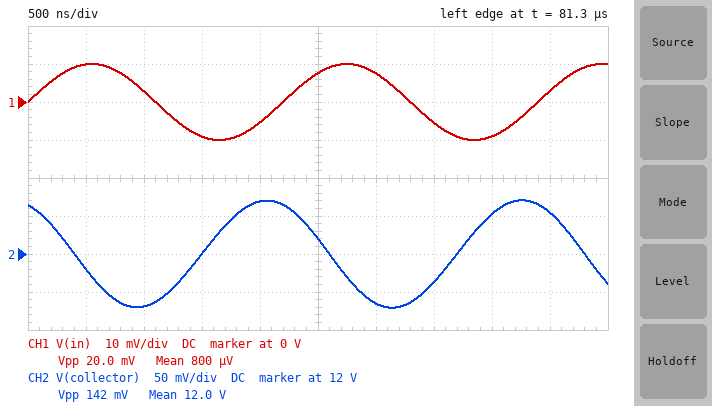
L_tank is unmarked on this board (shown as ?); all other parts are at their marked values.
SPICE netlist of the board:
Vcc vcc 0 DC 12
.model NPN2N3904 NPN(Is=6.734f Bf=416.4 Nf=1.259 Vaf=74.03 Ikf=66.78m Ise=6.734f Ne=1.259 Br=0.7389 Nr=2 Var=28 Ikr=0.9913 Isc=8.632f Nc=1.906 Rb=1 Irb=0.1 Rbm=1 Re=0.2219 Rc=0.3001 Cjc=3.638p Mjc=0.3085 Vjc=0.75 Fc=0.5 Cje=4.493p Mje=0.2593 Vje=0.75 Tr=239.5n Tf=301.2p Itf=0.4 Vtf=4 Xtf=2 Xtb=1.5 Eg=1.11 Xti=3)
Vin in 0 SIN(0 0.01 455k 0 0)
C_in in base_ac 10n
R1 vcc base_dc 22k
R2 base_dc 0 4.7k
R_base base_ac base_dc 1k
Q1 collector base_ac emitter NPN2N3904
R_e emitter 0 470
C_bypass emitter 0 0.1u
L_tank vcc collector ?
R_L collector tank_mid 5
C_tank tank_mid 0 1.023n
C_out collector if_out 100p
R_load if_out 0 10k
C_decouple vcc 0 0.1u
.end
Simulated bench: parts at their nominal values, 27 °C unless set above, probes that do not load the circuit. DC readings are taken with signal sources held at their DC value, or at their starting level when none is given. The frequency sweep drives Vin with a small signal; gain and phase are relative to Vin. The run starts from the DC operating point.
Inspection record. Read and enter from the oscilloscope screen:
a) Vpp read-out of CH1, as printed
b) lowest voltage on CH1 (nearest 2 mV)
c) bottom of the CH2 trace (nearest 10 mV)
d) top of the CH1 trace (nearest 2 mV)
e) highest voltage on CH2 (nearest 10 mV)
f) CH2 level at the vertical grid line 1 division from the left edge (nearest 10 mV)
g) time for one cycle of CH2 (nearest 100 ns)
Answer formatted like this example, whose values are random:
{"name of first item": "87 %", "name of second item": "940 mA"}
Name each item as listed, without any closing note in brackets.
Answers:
{"Vpp read-out of CH1, as printed": "20.0 mV", "lowest voltage on CH1": "-10 mV", "bottom of the CH2 trace": "11.93 V", "top of the CH1 trace": "10 mV", "highest voltage on CH2": "12.07 V", "CH2 level at the vertical grid line 1 division from the left edge": "11.98 V", "time for one cycle of CH2": "2.2 µs"}
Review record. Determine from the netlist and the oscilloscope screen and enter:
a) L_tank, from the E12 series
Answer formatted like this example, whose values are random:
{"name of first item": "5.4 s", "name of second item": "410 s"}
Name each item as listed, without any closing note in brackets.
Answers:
{"L_tank, from the E12 series": "180 µH"}
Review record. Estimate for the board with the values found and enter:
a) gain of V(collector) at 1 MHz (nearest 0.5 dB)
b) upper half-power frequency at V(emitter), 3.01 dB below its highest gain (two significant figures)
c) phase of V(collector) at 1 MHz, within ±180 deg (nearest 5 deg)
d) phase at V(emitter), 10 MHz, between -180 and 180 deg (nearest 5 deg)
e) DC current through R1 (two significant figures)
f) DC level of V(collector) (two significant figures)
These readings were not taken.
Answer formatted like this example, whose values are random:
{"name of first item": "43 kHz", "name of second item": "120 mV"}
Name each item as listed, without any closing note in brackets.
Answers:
{"gain of V(collector) at 1 MHz": "2.5 dB", "upper half-power frequency at V(emitter), 3.01 dB below its highest gain": "140 kHz", "phase of V(collector) at 1 MHz, within ±180 deg": "100 deg", "phase at V(emitter), 10 MHz, between -180 and 180 deg": "-85 deg", "DC current through R1": "490 µA", "DC level of V(collector)": "12 V"}
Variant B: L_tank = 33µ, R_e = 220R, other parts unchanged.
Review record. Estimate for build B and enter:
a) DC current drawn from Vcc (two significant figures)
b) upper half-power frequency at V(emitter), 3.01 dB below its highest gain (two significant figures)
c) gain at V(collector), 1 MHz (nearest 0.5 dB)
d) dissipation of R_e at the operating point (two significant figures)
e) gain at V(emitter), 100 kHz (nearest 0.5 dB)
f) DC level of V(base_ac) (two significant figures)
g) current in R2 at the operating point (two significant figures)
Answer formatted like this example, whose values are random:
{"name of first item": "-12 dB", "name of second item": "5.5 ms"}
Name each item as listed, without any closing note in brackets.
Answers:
{"DC current drawn from Vcc": "770 µA", "upper half-power frequency at V(emitter), 3.01 dB below its highest gain": "160 kHz", "gain at V(collector), 1 MHz": "14.0 dB", "dissipation of R_e at the operating point": "60 µW", "gain at V(emitter), 100 kHz": "-17.0 dB", "DC level of V(base_ac)": "910 mV", "current in R2 at the operating point": "250 µA"}
